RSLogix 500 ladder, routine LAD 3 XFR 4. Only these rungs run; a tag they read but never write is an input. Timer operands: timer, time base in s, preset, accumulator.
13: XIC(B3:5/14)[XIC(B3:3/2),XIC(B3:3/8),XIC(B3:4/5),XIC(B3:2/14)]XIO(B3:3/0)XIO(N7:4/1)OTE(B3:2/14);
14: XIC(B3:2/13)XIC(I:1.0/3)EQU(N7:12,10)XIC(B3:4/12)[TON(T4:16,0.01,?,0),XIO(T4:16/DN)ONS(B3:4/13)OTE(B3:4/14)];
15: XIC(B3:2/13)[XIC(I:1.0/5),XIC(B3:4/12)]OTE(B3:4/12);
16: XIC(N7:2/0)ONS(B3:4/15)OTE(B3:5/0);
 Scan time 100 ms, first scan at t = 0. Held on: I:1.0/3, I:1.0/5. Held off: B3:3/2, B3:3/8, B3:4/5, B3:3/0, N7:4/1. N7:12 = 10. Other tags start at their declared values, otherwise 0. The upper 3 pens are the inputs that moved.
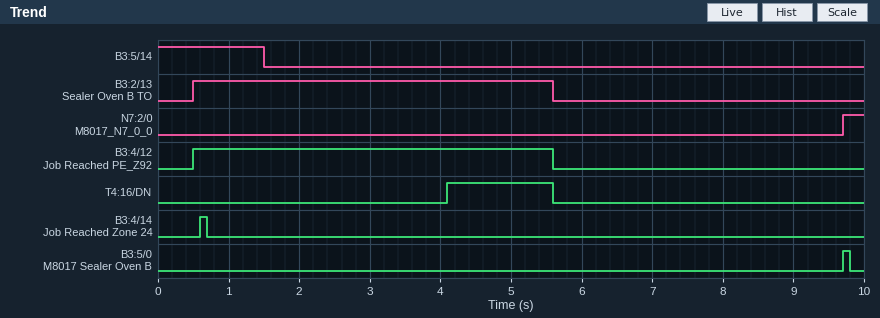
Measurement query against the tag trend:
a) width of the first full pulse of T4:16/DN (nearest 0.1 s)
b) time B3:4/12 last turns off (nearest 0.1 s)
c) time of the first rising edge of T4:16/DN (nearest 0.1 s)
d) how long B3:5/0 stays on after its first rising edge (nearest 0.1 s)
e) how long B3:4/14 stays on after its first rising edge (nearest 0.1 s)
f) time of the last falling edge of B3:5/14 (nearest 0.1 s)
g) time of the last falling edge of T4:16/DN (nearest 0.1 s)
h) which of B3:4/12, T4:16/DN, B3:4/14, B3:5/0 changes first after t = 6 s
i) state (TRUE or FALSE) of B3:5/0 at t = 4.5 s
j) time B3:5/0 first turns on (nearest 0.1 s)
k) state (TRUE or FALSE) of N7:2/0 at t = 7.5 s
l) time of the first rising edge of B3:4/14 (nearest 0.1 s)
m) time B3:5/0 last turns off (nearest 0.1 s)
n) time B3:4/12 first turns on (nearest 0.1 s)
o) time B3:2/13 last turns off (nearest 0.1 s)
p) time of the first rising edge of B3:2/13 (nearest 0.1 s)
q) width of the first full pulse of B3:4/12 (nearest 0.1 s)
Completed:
1.5 s
5.6 s
4.1 s
0.1 s
0.1 s
1.5 s
5.6 s
B3:5/0
FALSE
9.7 s
FALSE
0.6 s
9.8 s
0.5 s
5.6 s
0.5 s
5.1 s
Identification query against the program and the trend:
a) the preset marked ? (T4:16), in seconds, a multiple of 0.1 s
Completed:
3.5 s
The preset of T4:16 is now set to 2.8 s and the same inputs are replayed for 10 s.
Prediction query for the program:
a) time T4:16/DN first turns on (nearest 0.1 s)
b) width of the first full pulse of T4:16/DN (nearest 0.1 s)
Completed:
3.4 s
2.2 s
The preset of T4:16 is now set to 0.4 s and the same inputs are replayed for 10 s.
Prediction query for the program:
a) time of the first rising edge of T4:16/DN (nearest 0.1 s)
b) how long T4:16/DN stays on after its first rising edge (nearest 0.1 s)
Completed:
1.0 s
4.6 s
